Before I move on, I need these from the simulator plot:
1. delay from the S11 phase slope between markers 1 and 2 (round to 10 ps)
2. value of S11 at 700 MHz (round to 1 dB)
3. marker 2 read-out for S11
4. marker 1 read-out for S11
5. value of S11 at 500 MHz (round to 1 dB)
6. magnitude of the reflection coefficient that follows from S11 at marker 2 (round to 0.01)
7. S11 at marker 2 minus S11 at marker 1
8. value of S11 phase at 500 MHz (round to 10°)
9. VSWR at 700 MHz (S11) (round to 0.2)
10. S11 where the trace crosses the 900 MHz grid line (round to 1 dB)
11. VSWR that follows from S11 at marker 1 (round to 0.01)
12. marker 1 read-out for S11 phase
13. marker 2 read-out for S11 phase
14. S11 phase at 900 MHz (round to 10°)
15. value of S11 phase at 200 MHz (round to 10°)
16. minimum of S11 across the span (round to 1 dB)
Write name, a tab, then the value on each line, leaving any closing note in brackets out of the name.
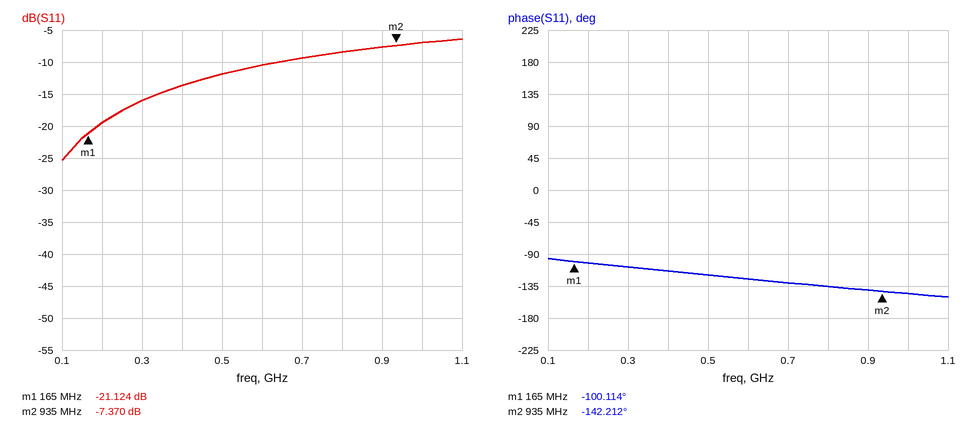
delay from the S11 phase slope between markers 1 and 2	150 ps
value of S11 at 700 MHz	-9 dB
marker 2 read-out for S11	-7.370 dB
marker 1 read-out for S11	-21.124 dB
value of S11 at 500 MHz	-12 dB
magnitude of the reflection coefficient that follows from S11 at marker 2	0.43
S11 at marker 2 minus S11 at marker 1	13.754 dB
value of S11 phase at 500 MHz	-120°
VSWR at 700 MHz (S11)	2.0
S11 where the trace crosses the 900 MHz grid line	-8 dB
VSWR that follows from S11 at marker 1	1.19
marker 1 read-out for S11 phase	-100.114°
marker 2 read-out for S11 phase	-142.212°
S11 phase at 900 MHz	-140°
value of S11 phase at 200 MHz	-100°
minimum of S11 across the span	-25 dB
